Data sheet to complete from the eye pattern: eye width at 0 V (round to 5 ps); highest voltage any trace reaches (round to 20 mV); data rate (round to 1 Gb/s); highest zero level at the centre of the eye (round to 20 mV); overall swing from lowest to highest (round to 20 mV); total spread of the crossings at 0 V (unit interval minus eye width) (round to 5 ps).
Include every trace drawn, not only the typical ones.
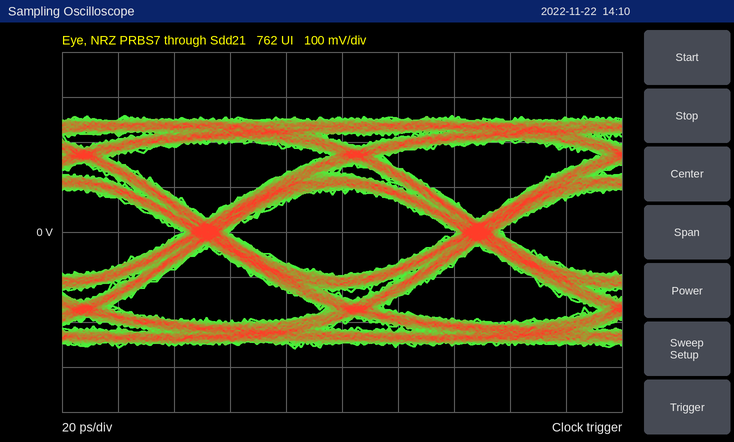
80 ps
260 mV
10 Gb/s
-100 mV
520 mV
15 ps
